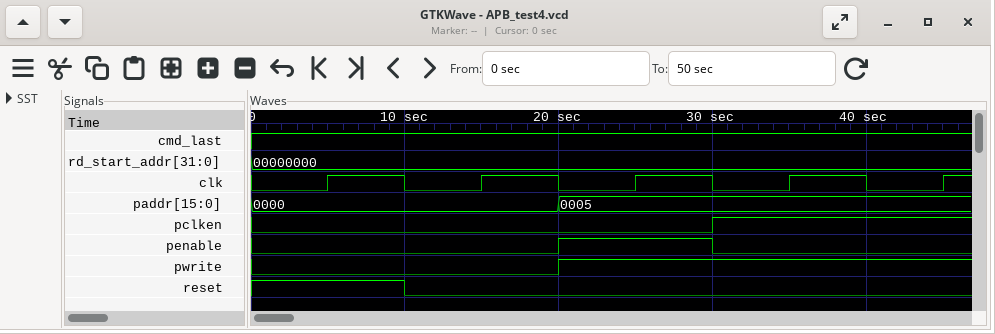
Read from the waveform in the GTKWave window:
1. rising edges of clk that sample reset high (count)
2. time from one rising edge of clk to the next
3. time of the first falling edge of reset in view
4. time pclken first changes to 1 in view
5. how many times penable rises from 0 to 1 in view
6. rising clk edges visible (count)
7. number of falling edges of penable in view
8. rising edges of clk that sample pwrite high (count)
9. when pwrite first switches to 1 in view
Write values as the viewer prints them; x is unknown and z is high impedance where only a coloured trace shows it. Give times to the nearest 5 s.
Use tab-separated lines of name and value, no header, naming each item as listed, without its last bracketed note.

rising edges of clk that sample reset high	1
time from one rising edge of clk to the next	10 s
time of the first falling edge of reset in view	10 s
time pclken first changes to 1 in view	30 s
how many times penable rises from 0 to 1 in view	1
rising clk edges visible	5
number of falling edges of penable in view	1
rising edges of clk that sample pwrite high	3
when pwrite first switches to 1 in view	20 s
